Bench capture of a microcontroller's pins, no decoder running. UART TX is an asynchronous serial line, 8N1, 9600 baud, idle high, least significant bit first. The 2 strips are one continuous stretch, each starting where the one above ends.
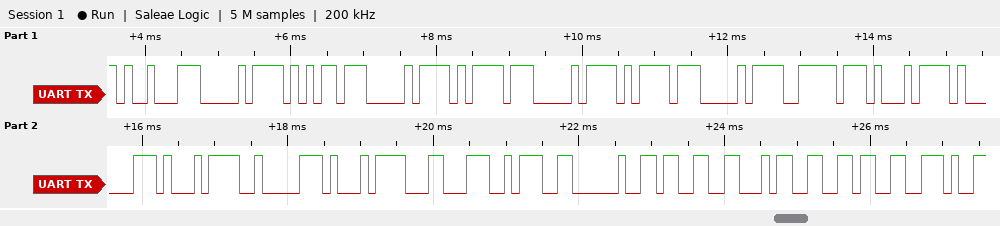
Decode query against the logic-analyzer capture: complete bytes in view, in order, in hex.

89 D0 B5 D0 BD D0 BD D0 BE D1 81 D1 82 D1 8C 3A 20 33 34 36 2E
